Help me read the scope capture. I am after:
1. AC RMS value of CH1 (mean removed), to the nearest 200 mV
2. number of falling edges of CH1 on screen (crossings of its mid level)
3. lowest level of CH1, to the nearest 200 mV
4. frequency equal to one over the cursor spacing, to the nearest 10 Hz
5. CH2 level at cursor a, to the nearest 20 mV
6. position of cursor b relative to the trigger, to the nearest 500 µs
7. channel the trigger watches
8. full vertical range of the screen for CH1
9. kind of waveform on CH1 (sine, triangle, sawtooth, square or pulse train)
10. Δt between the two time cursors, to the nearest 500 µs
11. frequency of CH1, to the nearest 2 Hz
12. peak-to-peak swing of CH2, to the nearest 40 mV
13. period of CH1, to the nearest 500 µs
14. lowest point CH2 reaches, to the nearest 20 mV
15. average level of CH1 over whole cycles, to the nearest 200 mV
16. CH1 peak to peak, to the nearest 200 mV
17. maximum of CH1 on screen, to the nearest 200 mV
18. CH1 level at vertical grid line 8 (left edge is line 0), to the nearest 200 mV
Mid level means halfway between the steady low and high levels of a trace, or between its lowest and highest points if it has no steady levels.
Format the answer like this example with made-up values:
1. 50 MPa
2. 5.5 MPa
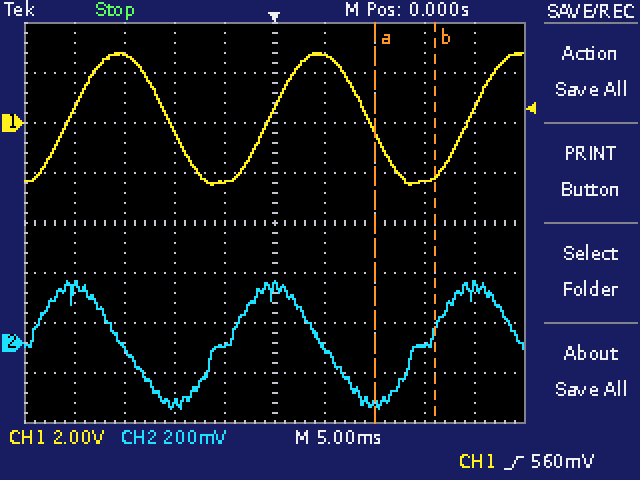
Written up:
1. 1.8 V
2. 2
3. -2.4 V
4. 170 Hz
5. -240 mV
6. +16.0 ms
7. CH1
8. 16 V
9. sine
10. 6.0 ms
11. 50 Hz
12. 520 mV
13. 20.0 ms
14. -260 mV
15. 200 mV
16. 5.2 V
17. 2.8 V
18. -2.4 V
